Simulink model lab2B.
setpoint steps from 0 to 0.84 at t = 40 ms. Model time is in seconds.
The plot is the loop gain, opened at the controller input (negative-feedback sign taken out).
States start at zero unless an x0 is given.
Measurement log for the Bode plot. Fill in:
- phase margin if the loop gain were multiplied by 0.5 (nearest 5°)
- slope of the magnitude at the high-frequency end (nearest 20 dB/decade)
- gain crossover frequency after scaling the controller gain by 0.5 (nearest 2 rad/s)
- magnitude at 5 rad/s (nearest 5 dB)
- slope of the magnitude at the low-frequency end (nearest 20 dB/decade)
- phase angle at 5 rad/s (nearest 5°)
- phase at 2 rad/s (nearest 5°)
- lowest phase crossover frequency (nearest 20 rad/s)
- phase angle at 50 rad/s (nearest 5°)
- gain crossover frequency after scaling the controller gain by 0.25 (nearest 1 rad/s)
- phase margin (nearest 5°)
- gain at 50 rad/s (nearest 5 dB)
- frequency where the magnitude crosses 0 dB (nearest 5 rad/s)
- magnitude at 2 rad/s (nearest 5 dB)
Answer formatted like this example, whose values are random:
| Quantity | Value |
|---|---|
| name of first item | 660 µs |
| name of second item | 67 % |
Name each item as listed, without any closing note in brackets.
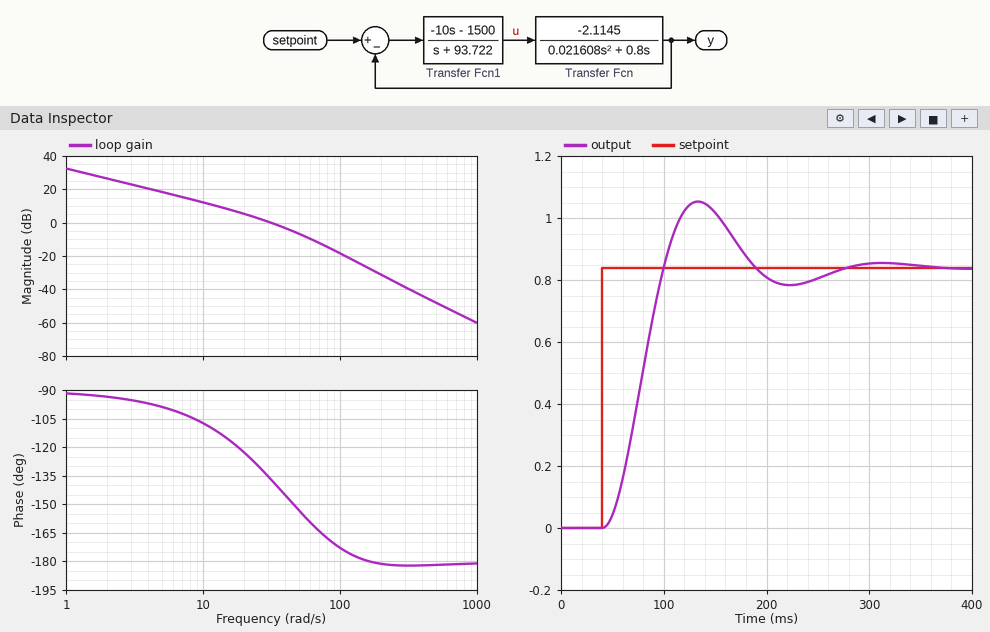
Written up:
| Quantity | Value |
|---|---|
| phase margin if the loop gain were multiplied by 0.5 | 60° |
| slope of the magnitude at the high-frequency end | -40 dB/decade |
| gain crossover frequency after scaling the controller gain by 0.5 | 18 rad/s |
| magnitude at 5 rad/s | 20 dB |
| slope of the magnitude at the low-frequency end | -20 dB/decade |
| phase angle at 5 rad/s | -100° |
| phase at 2 rad/s | -95° |
| lowest phase crossover frequency | 160 rad/s |
| phase angle at 50 rad/s | -155° |
| gain crossover frequency after scaling the controller gain by 0.25 | 10 rad/s |
| phase margin | 45° |
| gain at 50 rad/s | -5 dB |
| frequency where the magnitude crosses 0 dB | 30 rad/s |
| magnitude at 2 rad/s | 25 dB |
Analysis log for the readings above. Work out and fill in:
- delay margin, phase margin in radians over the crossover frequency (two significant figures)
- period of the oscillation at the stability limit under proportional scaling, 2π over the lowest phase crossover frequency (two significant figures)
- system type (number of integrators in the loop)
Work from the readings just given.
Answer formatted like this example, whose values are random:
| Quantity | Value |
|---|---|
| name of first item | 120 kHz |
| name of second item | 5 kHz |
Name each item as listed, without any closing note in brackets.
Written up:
| Quantity | Value |
|---|---|
| delay margin, phase margin in radians over the crossover frequency | 0.026 s |
| period of the oscillation at the stability limit under proportional scaling, 2π over the lowest phase crossover frequency | 0.039 s |
| system type | 1 |
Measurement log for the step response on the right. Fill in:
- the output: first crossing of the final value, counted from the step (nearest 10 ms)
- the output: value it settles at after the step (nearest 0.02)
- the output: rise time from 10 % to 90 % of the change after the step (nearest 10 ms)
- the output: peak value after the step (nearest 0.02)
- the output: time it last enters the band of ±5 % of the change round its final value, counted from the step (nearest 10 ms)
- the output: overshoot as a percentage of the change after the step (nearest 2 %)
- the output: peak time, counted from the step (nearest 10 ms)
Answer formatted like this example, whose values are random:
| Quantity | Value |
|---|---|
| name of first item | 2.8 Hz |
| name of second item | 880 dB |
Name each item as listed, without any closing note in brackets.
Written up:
| Quantity | Value |
|---|---|
| the output: first crossing of the final value, counted from the step | 60 ms |
| the output: value it settles at after the step | 0.84 |
| the output: rise time from 10 % to 90 % of the change after the step | 40 ms |
| the output: peak value after the step | 1.06 |
| the output: time it last enters the band of ±5 % of the change round its final value, counted from the step | 200 ms |
| the output: overshoot as a percentage of the change after the step | 26 % |
| the output: peak time, counted from the step | 90 ms |
